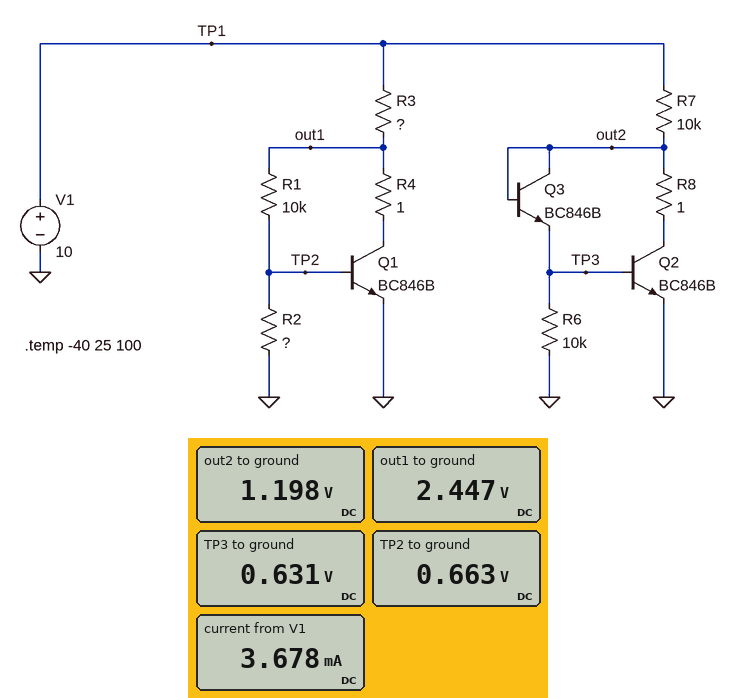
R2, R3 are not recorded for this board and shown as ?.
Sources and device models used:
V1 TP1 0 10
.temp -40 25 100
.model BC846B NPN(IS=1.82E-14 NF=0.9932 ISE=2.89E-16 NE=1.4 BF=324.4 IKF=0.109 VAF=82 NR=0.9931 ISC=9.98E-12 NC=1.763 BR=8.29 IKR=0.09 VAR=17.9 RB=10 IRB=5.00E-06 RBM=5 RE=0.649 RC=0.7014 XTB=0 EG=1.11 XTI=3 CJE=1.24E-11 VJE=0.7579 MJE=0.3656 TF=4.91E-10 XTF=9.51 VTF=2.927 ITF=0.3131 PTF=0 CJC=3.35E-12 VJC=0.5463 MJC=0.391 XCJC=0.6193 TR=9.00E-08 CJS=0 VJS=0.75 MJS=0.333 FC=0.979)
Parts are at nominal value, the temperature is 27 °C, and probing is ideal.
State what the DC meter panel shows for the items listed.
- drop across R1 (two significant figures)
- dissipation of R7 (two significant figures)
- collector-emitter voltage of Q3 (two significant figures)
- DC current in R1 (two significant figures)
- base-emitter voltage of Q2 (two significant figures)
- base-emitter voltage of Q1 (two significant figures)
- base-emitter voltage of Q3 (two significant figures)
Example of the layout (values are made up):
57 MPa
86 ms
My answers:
1.8 V
7.7 mW
570 mV
180 µA
630 mV
660 mV
570 mV
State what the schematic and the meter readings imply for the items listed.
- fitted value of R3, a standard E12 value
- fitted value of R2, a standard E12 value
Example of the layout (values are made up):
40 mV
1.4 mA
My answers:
2.7 kΩ
3.9 kΩ
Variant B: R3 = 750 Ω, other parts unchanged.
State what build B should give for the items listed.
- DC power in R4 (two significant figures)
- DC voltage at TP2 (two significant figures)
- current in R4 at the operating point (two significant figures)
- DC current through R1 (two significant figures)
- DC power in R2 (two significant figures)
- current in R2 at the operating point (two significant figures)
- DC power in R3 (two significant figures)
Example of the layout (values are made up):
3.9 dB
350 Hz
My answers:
88 µW
700 mV
9.4 mA
210 µA
130 µW
180 µA
69 mW
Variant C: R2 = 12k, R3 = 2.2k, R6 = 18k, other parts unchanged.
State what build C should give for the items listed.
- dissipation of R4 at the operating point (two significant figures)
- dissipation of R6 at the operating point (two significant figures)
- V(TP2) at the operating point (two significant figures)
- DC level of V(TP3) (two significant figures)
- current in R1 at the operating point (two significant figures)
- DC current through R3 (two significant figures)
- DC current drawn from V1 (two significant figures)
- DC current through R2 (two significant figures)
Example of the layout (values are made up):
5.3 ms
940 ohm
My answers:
15 µW
22 µW
670 mV
630 mV
69 µA
3.9 mA
4.8 mA
56 µA
